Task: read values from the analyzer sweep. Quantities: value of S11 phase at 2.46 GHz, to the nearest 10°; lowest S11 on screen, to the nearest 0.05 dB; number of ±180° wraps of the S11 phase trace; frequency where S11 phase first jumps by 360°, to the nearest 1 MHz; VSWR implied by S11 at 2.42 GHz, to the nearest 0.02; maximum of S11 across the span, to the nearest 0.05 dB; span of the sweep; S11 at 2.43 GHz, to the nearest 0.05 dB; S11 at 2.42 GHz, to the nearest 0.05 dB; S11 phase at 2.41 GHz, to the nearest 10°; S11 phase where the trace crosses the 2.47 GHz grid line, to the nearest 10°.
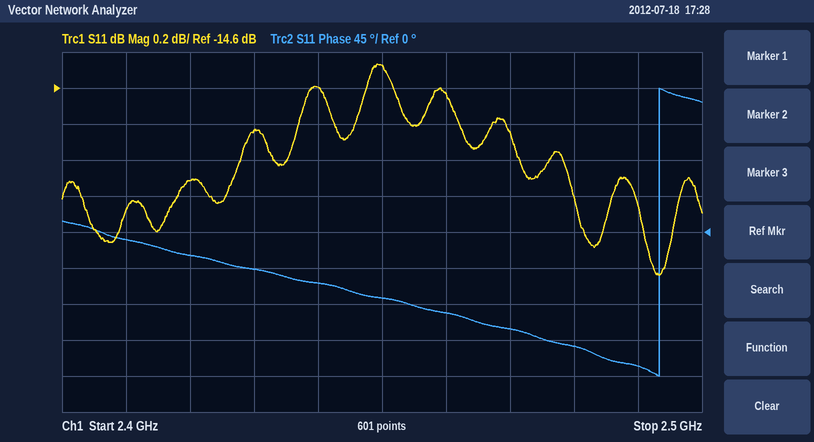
-100°
-15.65 dB
1
2.493 GHz
1.42
-14.45 dB
100 MHz
-14.85 dB
-15.10 dB
-10°
-120°
